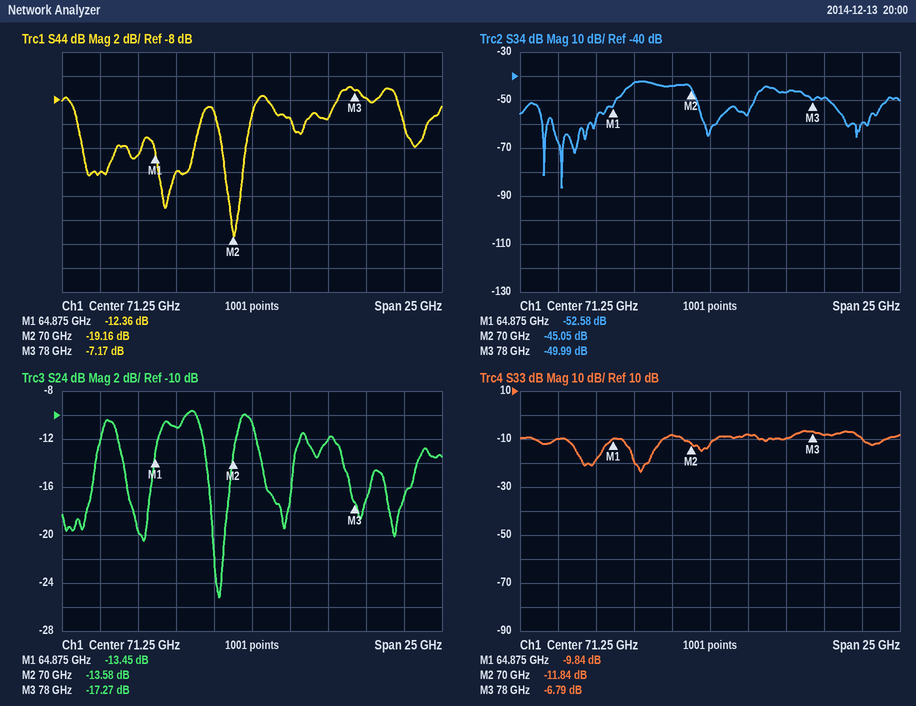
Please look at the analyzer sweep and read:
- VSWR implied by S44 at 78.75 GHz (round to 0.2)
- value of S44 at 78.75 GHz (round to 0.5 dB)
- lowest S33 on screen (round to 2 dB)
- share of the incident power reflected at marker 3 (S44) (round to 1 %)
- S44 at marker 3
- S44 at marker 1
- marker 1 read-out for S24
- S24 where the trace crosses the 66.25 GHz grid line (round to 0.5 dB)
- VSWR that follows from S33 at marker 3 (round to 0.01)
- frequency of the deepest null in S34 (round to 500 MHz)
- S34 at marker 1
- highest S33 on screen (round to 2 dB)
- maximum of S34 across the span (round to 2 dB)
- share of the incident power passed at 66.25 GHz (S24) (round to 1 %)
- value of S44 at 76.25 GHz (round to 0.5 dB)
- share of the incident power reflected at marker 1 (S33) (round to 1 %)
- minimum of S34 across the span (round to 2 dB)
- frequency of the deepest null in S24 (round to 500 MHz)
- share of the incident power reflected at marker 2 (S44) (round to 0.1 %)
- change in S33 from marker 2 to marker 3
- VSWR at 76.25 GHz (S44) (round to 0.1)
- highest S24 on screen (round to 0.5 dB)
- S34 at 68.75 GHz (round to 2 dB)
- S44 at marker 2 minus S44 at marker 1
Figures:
2.4
-8.0 dB
-24 dB
19 %
-7.17 dB
-12.36 dB
-13.45 dB
-11.0 dB
2.69
61.5 GHz
-52.58 dB
-6 dB
-42 dB
8 %
-9.5 dB
10 %
-86 dB
69.0 GHz
1.2 %
5.05 dB
2.0
-9.5 dB
-44 dB
-6.80 dB
